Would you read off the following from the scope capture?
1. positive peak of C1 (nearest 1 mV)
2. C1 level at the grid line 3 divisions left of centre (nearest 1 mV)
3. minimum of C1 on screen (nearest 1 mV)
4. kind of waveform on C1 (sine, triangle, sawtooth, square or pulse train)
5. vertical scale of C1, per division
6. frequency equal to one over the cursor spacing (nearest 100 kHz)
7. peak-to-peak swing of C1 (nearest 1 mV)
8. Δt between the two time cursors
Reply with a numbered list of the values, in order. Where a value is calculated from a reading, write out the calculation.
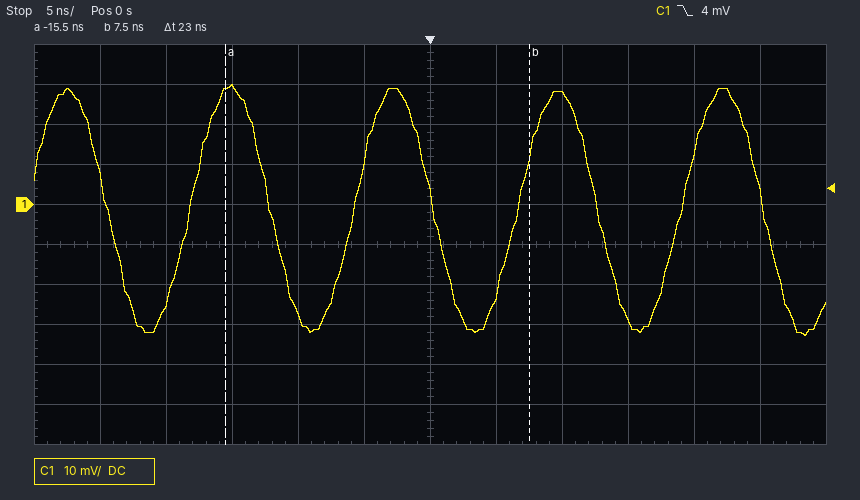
1. 30 mV
2. 29 mV
3. -33 mV
4. sine
5. 10 mV
6. 1 / 23 ns ≈ 43.5 MHz
7. 30 mV − (-33 mV) = 63 mV
8. 23 ns
